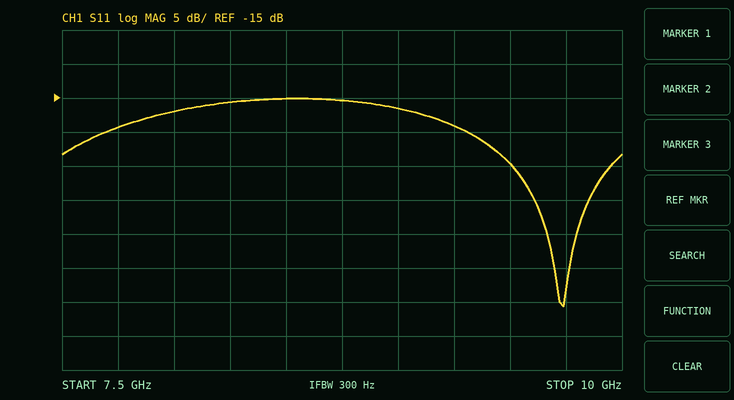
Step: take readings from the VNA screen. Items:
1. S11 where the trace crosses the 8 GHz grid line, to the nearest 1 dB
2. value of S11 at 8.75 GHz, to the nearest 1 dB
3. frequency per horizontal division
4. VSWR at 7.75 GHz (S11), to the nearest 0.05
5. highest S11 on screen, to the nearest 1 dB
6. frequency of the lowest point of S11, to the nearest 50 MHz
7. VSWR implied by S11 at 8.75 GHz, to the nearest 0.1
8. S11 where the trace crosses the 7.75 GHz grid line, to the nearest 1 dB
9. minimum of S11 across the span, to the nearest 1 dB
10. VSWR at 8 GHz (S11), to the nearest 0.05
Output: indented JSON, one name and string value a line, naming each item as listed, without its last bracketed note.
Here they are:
{
  "S11 where the trace crosses the 8 GHz grid line, to the nearest 1 dB": "-17 dB",
  "value of S11 at 8.75 GHz, to the nearest 1 dB": "-15 dB",
  "frequency per horizontal division": "250 MHz",
  "VSWR at 7.75 GHz (S11), to the nearest 0.05": "1.25",
  "highest S11 on screen, to the nearest 1 dB": "-15 dB",
  "frequency of the lowest point of S11, to the nearest 50 MHz": "9.75 GHz",
  "VSWR implied by S11 at 8.75 GHz, to the nearest 0.1": "1.4",
  "S11 where the trace crosses the 7.75 GHz grid line, to the nearest 1 dB": "-19 dB",
  "minimum of S11 across the span, to the nearest 1 dB": "-46 dB",
  "VSWR at 8 GHz (S11), to the nearest 0.05": "1.35"
}
